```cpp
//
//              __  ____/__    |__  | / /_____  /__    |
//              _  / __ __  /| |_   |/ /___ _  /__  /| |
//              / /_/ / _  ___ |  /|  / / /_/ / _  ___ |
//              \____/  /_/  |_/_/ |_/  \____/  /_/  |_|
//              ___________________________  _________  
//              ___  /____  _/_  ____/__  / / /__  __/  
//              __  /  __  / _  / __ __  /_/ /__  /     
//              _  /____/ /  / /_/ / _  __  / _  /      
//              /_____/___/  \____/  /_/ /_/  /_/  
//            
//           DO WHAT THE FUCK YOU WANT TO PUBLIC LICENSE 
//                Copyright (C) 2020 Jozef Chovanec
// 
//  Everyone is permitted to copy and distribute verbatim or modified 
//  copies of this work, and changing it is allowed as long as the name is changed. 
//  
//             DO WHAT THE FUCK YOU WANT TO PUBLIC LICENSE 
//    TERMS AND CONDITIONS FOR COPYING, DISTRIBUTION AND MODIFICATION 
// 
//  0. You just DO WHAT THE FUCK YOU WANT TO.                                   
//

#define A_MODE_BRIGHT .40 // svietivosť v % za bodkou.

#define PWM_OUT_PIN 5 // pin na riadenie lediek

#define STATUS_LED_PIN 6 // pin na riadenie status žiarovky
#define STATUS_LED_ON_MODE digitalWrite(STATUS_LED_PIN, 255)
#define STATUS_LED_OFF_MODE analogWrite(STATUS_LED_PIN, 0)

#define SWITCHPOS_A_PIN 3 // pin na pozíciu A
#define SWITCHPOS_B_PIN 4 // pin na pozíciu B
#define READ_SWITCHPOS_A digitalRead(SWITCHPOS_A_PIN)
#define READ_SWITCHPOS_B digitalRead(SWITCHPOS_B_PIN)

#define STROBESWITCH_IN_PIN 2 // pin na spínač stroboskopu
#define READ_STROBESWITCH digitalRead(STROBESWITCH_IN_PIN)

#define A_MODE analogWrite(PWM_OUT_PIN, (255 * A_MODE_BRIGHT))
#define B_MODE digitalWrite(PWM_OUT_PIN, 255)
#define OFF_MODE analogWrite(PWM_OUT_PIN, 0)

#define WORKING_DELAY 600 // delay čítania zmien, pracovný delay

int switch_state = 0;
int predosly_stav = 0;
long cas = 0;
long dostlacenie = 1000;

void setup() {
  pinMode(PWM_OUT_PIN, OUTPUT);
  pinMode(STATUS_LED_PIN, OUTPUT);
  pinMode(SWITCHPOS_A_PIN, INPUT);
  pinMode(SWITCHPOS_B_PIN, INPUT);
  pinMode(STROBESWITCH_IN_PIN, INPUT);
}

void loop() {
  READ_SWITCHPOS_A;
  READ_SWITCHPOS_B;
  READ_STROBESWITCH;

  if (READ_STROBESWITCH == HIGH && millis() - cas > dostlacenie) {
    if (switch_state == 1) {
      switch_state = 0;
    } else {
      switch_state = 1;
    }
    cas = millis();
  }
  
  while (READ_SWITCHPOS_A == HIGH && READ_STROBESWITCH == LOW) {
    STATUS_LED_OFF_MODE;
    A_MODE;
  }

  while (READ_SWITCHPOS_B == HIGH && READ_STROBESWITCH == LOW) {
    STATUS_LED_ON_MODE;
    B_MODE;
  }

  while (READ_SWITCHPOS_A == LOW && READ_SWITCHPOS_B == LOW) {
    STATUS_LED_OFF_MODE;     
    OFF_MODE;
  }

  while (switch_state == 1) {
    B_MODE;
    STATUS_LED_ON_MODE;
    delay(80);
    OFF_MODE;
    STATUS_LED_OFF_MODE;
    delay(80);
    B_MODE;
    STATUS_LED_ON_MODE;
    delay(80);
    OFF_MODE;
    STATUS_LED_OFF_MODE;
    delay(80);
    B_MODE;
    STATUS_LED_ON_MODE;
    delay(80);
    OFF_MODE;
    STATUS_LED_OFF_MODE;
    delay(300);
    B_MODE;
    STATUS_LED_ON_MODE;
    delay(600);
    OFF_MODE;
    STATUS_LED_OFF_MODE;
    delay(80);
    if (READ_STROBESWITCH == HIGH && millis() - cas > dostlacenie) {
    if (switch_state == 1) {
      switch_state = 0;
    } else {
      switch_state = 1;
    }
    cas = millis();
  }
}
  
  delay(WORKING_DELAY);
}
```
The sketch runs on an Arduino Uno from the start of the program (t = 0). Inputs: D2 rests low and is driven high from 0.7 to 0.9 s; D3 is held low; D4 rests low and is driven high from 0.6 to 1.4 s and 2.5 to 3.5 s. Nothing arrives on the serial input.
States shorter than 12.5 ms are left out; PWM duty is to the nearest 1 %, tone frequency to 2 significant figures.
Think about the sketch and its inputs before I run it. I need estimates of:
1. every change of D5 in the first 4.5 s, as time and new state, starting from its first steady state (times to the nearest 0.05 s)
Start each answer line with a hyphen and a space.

- 0 s low; 1.2 s high; 1.4 s low; 3.1 s high; 3.5 s low
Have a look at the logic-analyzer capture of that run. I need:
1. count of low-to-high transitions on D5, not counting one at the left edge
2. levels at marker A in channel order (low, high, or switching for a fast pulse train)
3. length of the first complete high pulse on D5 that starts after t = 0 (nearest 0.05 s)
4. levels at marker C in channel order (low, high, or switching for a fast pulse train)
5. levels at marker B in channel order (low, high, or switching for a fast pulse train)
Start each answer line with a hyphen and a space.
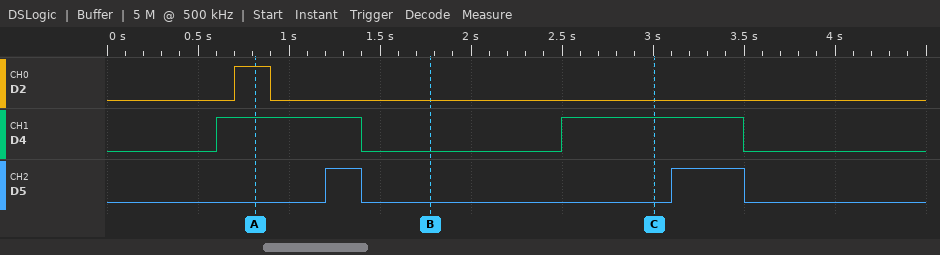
- 2
- D2 high, D4 high, D5 low
- 0.20 s
- D2 low, D4 high, D5 low
- D2 low, D4 low, D5 low
